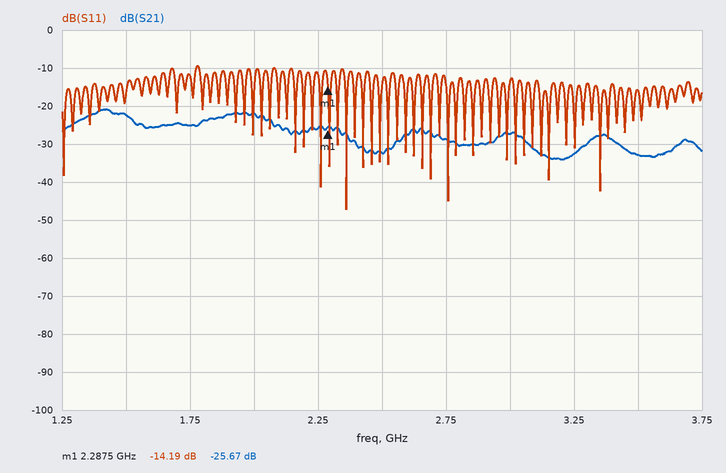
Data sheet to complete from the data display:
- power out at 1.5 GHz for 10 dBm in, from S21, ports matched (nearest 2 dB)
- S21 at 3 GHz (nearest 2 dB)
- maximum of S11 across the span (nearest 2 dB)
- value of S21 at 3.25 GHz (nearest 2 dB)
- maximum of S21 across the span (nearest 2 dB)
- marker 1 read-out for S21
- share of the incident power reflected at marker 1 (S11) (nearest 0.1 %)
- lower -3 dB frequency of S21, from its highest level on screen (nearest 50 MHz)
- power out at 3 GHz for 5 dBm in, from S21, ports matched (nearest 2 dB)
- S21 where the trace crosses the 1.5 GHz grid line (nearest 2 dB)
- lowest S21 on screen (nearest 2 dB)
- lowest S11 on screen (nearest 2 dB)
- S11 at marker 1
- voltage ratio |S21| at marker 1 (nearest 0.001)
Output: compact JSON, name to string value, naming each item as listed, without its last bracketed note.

{"power out at 1.5 GHz for 10 dBm in, from S21, ports matched": "-12 dBm", "S21 at 3 GHz": "-28 dB", "maximum of S11 across the span": "-10 dB", "value of S21 at 3.25 GHz": "-32 dB", "maximum of S21 across the span": "-20 dB", "marker 1 read-out for S21": "-25.67 dB", "share of the incident power reflected at marker 1 (S11)": "3.8 %", "lower -3 dB frequency of S21, from its highest level on screen": "1.30 GHz", "power out at 3 GHz for 5 dBm in, from S21, ports matched": "-22 dBm", "S21 where the trace crosses the 1.5 GHz grid line": "-22 dB", "lowest S21 on screen": "-34 dB", "lowest S11 on screen": "-48 dB", "S11 at marker 1": "-14.19 dB", "voltage ratio |S21| at marker 1": "0.052"}
